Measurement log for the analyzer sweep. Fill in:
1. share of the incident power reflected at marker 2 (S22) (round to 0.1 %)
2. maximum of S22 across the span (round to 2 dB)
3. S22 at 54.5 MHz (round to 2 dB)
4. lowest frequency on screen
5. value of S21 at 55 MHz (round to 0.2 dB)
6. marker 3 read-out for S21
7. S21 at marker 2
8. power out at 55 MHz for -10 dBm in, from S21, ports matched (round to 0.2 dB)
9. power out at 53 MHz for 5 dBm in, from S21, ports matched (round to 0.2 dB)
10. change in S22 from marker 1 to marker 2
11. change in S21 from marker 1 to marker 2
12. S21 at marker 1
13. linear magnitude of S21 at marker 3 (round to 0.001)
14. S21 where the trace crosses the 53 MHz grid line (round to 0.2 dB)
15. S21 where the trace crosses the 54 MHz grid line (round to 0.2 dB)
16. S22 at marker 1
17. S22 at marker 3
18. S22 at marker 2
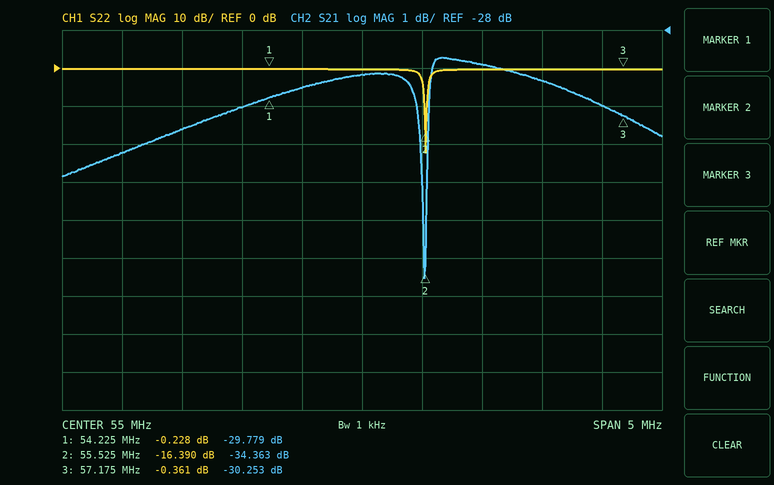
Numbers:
2.3 %
0 dB
0 dB
52.5 MHz
-29.2 dB
-30.253 dB
-34.363 dB
-39.2 dBm
-26.2 dBm
-16.162 dB
-4.584 dB
-29.779 dB
0.031
-31.2 dB
-30.0 dB
-0.228 dB
-0.361 dB
-16.390 dB
